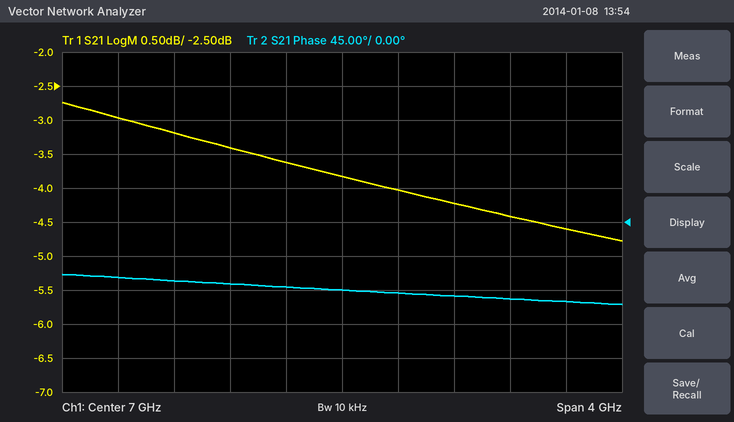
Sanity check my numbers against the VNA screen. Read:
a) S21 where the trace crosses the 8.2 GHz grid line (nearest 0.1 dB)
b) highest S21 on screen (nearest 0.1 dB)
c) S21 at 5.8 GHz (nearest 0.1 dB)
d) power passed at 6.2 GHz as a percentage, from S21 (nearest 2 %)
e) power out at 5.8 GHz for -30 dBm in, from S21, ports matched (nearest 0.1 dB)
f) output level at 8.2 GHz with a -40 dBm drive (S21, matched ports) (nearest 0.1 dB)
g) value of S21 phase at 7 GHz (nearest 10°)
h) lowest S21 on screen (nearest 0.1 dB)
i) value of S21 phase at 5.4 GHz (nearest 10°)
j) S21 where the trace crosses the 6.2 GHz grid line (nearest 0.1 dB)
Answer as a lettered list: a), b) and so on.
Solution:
a) -4.4 dB
b) -2.7 dB
c) -3.2 dB
d) 46 %
e) -33.2 dBm
f) -44.4 dBm
g) -90°
h) -4.8 dB
i) -70°
j) -3.4 dB
